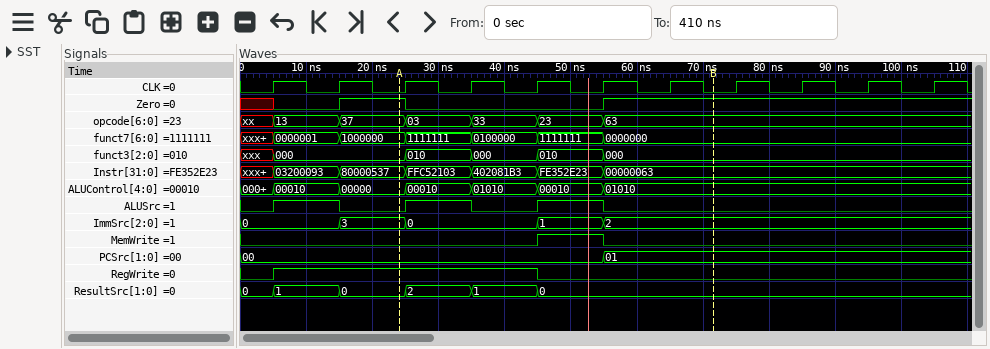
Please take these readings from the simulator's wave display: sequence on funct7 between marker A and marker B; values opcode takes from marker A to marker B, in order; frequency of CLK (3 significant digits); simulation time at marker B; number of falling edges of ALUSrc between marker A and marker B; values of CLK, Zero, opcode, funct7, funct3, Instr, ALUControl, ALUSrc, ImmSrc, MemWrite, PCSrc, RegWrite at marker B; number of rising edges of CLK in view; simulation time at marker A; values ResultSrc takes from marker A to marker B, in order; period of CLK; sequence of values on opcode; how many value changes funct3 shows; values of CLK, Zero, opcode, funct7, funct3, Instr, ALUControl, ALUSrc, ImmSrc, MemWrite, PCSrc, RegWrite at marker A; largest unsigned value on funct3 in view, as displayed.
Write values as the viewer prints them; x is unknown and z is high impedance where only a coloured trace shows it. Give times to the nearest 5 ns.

1000000, 1111111, 0100000, 1111111, 0000000
37, 03, 33, 23, 63
100 MHz
70 ns
2
CLK=0, Zero=1, opcode=63, funct7=0000000, funct3=000, Instr=00000063, ALUControl=01010, ALUSrc=0, ImmSrc=2, MemWrite=0, PCSrc=01, RegWrite=0
11
25 ns
0, 2, 1, 0
10 ns
xx, 13, 37, 03, 33, 23, 63
5
CLK=0, Zero=1, opcode=37, funct7=1000000, funct3=000, Instr=80000537, ALUControl=00000, ALUSrc=0, ImmSrc=3, MemWrite=0, PCSrc=00, RegWrite=1
010
